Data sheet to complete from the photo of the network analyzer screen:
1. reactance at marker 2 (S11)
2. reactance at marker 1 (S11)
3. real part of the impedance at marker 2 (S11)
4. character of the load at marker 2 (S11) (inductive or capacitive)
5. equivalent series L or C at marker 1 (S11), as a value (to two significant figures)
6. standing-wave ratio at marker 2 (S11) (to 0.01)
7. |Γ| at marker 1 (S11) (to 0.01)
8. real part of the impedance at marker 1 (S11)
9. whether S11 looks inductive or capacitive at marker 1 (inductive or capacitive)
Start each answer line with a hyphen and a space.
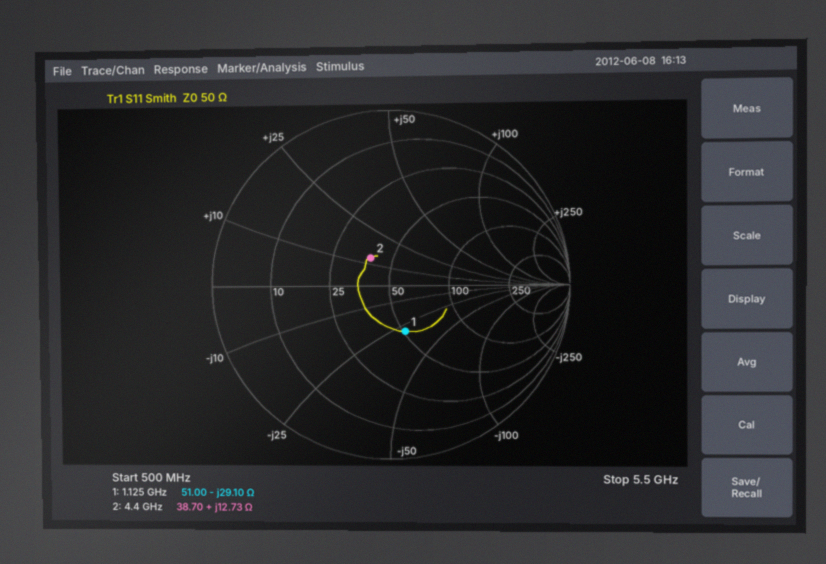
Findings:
- +12.73 Ω
- -29.10 Ω
- 38.70 Ω
- inductive
- 4.9 pF
- 1.47
- 0.28
- 51.00 Ω
- capacitive
